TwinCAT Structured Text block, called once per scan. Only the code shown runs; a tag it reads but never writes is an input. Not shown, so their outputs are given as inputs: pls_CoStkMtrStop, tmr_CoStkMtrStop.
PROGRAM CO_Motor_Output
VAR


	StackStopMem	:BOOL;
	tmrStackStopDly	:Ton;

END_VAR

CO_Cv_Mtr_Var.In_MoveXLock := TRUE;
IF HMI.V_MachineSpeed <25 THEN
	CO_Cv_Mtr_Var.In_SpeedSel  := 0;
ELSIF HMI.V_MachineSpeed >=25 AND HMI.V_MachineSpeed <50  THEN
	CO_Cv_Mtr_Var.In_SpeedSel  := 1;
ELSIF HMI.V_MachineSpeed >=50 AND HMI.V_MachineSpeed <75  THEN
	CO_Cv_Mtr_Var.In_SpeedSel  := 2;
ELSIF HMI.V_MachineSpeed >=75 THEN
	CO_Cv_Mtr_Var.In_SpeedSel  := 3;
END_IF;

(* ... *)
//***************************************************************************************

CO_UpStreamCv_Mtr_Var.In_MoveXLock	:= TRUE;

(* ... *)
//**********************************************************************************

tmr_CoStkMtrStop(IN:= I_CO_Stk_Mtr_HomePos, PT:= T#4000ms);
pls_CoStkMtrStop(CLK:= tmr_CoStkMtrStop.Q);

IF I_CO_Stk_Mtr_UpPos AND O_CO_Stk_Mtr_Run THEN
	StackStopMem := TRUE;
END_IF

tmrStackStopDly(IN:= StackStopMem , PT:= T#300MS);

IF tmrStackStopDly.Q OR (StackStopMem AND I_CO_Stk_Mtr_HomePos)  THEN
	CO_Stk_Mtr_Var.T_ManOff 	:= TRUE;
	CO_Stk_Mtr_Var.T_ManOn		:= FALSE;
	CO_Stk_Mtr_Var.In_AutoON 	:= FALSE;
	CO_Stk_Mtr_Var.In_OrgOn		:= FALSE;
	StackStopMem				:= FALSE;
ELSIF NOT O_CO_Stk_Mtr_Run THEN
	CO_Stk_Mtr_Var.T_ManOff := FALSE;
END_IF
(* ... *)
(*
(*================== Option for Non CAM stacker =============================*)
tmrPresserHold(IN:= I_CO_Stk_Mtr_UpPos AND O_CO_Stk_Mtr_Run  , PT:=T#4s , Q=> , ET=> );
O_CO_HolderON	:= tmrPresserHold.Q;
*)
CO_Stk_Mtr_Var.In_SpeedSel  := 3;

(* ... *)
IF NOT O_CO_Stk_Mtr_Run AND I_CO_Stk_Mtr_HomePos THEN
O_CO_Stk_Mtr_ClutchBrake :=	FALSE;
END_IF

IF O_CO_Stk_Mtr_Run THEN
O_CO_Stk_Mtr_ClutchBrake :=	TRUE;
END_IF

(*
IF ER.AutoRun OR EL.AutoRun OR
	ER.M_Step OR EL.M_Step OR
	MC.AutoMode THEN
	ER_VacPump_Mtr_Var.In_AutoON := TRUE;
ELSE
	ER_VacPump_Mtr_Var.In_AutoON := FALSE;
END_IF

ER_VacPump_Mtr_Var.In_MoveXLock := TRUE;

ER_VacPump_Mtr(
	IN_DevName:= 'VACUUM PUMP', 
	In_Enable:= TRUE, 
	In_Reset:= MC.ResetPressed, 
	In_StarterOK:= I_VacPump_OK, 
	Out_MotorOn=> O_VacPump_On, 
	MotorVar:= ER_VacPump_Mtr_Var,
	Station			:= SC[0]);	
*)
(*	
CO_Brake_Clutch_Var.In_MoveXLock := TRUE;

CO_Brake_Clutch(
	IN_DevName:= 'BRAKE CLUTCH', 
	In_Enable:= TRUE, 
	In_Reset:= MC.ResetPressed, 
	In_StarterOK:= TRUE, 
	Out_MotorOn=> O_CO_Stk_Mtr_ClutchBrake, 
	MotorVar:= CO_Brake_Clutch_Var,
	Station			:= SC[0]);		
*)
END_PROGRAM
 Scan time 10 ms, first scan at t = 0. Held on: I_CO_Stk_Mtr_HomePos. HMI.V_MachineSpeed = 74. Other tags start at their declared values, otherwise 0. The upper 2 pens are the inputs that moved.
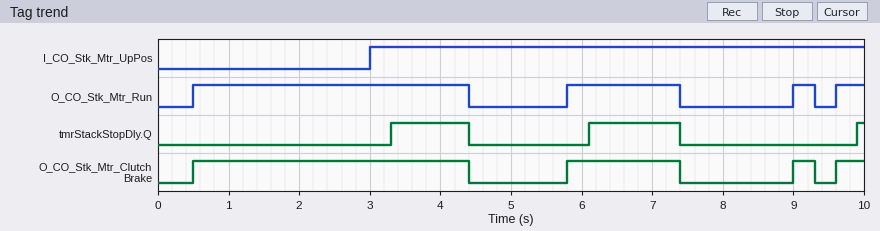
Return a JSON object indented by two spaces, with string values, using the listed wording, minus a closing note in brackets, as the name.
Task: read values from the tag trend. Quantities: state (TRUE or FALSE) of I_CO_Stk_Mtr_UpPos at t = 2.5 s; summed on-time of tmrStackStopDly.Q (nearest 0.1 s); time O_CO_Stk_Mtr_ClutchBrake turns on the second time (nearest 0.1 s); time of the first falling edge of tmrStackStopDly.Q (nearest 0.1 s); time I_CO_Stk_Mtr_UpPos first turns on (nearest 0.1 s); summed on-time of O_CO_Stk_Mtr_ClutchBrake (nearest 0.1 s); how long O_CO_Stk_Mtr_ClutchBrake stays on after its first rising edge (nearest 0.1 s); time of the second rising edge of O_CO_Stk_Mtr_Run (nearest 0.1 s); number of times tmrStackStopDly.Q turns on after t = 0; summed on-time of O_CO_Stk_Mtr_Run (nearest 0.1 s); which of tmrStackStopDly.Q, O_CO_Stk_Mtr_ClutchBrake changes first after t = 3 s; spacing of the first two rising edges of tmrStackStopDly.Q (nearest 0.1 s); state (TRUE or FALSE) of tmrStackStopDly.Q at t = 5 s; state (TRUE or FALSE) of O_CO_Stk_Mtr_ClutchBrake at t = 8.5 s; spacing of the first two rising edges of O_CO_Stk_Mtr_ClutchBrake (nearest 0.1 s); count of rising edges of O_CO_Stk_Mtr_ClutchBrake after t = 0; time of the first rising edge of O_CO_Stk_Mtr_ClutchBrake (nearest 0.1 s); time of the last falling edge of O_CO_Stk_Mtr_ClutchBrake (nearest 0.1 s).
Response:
{
  "state (TRUE or FALSE) of I_CO_Stk_Mtr_UpPos at t = 2.5 s": "FALSE",
  "summed on-time of tmrStackStopDly.Q": "2.5 s",
  "time O_CO_Stk_Mtr_ClutchBrake turns on the second time": "5.8 s",
  "time of the first falling edge of tmrStackStopDly.Q": "4.4 s",
  "time I_CO_Stk_Mtr_UpPos first turns on": "3.0 s",
  "summed on-time of O_CO_Stk_Mtr_ClutchBrake": "6.2 s",
  "how long O_CO_Stk_Mtr_ClutchBrake stays on after its first rising edge": "3.9 s",
  "time of the second rising edge of O_CO_Stk_Mtr_Run": "5.8 s",
  "number of times tmrStackStopDly.Q turns on after t = 0": "3",
  "summed on-time of O_CO_Stk_Mtr_Run": "6.2 s",
  "which of tmrStackStopDly.Q, O_CO_Stk_Mtr_ClutchBrake changes first after t = 3 s": "tmrStackStopDly.Q",
  "spacing of the first two rising edges of tmrStackStopDly.Q": "2.8 s",
  "state (TRUE or FALSE) of tmrStackStopDly.Q at t = 5 s": "FALSE",
  "state (TRUE or FALSE) of O_CO_Stk_Mtr_ClutchBrake at t = 8.5 s": "FALSE",
  "spacing of the first two rising edges of O_CO_Stk_Mtr_ClutchBrake": "5.3 s",
  "count of rising edges of O_CO_Stk_Mtr_ClutchBrake after t = 0": "4",
  "time of the first rising edge of O_CO_Stk_Mtr_ClutchBrake": "0.5 s",
  "time of the last falling edge of O_CO_Stk_Mtr_ClutchBrake": "9.3 s"
}
